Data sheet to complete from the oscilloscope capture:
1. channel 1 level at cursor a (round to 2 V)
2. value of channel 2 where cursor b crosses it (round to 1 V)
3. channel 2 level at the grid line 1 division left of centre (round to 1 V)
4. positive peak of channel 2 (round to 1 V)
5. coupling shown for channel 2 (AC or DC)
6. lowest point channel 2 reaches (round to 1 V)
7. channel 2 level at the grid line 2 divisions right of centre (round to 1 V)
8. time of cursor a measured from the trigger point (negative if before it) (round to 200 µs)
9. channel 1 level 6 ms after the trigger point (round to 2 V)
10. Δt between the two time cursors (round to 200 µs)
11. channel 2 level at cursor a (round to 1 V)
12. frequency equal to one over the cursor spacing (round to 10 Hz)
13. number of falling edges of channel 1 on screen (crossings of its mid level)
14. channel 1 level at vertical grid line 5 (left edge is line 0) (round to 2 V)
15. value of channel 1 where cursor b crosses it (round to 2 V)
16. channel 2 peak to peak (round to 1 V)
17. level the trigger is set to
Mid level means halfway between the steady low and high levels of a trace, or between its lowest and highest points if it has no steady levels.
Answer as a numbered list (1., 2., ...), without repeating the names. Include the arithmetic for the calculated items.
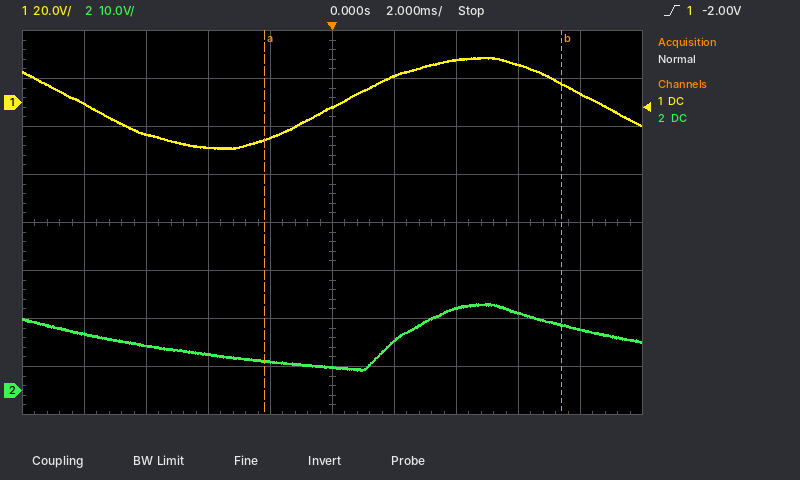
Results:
1. -16 V
2. 14 V
3. 6 V
4. 18 V
5. DC
6. 4 V
7. 17 V
8. -2.2 ms
9. 16 V
10. 9.6 ms
11. 6 V
12. 1 / 9.6 ms ≈ 100 Hz
13. 2
14. -2 V
15. 8 V
16. 18 V − (4 V) = 14 V
17. -2.00 V
